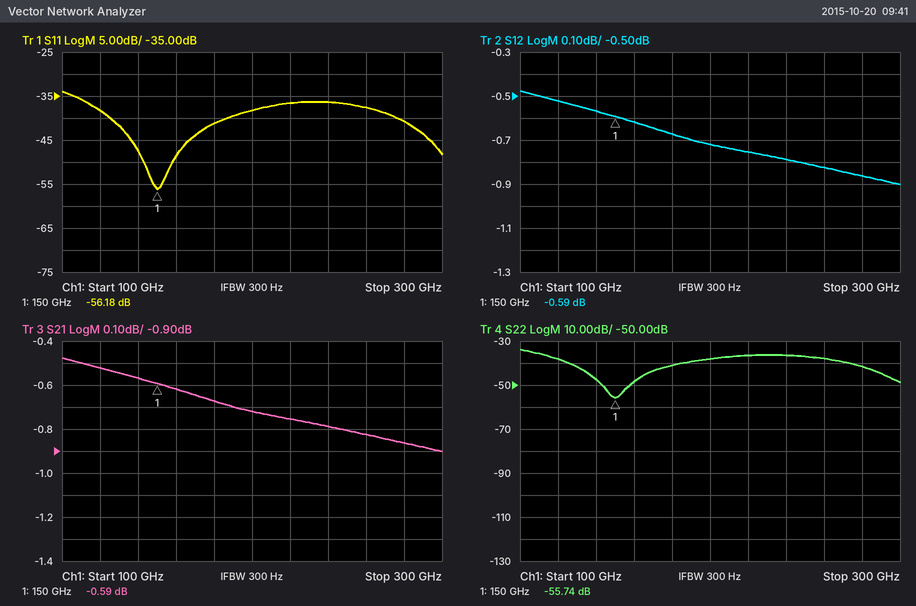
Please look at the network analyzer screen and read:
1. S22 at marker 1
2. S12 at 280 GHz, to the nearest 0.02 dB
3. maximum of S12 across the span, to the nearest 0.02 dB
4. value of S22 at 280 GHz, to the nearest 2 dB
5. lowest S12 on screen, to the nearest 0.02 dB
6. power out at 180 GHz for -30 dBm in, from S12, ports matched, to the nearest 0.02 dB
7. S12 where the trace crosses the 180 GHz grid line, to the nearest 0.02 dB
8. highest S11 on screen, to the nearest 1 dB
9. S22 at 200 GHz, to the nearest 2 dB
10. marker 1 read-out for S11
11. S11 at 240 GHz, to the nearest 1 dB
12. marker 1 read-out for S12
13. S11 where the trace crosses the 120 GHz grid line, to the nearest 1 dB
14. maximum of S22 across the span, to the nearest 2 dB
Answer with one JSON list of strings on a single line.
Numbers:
["-55.74 dB", "-0.86 dB", "-0.48 dB", "-42 dB", "-0.90 dB", "-30.68 dBm", "-0.68 dB", "-34 dB", "-38 dB", "-56.18 dB", "-36 dB", "-0.59 dB", "-38 dB", "-34 dB"]
